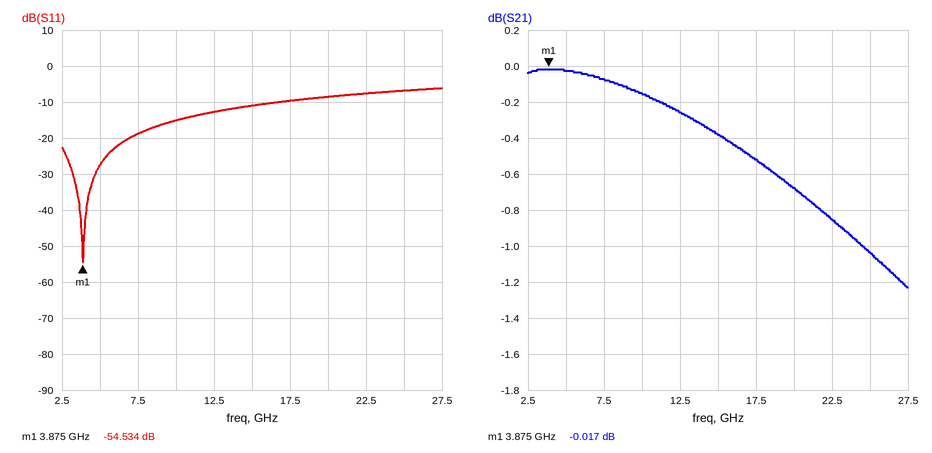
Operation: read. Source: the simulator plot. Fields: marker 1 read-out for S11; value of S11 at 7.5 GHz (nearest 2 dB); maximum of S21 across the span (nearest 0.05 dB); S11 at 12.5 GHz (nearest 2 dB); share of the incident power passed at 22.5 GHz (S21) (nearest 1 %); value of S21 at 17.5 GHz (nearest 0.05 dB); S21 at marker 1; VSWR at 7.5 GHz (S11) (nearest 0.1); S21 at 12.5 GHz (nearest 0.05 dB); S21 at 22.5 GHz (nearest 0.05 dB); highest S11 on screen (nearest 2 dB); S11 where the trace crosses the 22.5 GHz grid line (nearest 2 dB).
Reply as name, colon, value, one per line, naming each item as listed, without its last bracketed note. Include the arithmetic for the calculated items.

marker 1 read-out for S11: -54.534 dB
value of S11 at 7.5 GHz: -18 dB
maximum of S21 across the span: 0.00 dB
S11 at 12.5 GHz: -12 dB
share of the incident power passed at 22.5 GHz (S21): 10^(-0.85/10) ≈ 82 %
value of S21 at 17.5 GHz: -0.50 dB
S21 at marker 1: -0.017 dB
VSWR at 7.5 GHz (S11): |Γ| = 10^(-18/20) = 0.1259; VSWR = (1 + 0.1259)/(1 − 0.1259) ≈ 1.3
S21 at 12.5 GHz: -0.25 dB
S21 at 22.5 GHz: -0.85 dB
highest S11 on screen: -6 dB
S11 where the trace crosses the 22.5 GHz grid line: -8 dB
